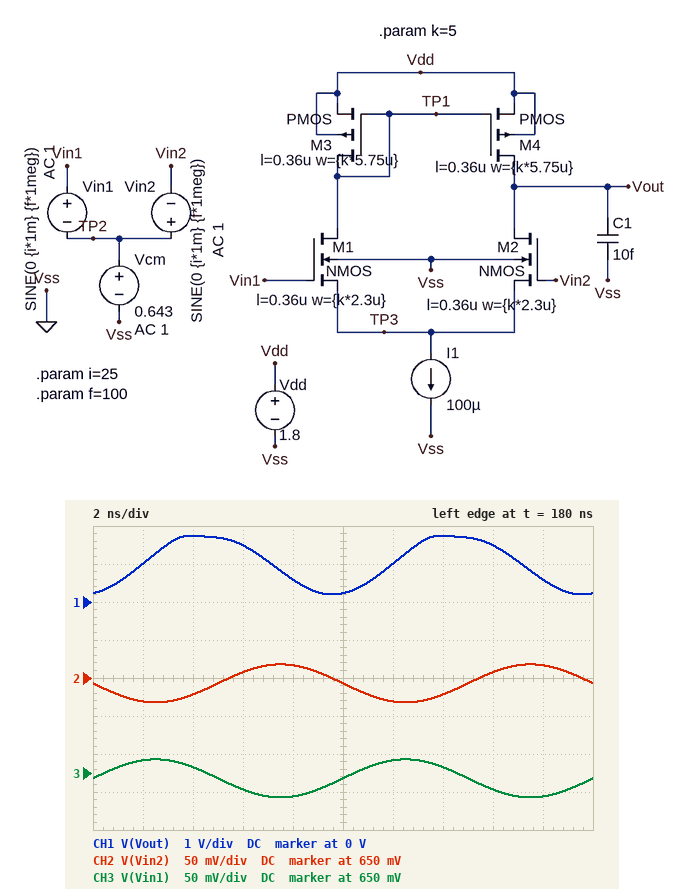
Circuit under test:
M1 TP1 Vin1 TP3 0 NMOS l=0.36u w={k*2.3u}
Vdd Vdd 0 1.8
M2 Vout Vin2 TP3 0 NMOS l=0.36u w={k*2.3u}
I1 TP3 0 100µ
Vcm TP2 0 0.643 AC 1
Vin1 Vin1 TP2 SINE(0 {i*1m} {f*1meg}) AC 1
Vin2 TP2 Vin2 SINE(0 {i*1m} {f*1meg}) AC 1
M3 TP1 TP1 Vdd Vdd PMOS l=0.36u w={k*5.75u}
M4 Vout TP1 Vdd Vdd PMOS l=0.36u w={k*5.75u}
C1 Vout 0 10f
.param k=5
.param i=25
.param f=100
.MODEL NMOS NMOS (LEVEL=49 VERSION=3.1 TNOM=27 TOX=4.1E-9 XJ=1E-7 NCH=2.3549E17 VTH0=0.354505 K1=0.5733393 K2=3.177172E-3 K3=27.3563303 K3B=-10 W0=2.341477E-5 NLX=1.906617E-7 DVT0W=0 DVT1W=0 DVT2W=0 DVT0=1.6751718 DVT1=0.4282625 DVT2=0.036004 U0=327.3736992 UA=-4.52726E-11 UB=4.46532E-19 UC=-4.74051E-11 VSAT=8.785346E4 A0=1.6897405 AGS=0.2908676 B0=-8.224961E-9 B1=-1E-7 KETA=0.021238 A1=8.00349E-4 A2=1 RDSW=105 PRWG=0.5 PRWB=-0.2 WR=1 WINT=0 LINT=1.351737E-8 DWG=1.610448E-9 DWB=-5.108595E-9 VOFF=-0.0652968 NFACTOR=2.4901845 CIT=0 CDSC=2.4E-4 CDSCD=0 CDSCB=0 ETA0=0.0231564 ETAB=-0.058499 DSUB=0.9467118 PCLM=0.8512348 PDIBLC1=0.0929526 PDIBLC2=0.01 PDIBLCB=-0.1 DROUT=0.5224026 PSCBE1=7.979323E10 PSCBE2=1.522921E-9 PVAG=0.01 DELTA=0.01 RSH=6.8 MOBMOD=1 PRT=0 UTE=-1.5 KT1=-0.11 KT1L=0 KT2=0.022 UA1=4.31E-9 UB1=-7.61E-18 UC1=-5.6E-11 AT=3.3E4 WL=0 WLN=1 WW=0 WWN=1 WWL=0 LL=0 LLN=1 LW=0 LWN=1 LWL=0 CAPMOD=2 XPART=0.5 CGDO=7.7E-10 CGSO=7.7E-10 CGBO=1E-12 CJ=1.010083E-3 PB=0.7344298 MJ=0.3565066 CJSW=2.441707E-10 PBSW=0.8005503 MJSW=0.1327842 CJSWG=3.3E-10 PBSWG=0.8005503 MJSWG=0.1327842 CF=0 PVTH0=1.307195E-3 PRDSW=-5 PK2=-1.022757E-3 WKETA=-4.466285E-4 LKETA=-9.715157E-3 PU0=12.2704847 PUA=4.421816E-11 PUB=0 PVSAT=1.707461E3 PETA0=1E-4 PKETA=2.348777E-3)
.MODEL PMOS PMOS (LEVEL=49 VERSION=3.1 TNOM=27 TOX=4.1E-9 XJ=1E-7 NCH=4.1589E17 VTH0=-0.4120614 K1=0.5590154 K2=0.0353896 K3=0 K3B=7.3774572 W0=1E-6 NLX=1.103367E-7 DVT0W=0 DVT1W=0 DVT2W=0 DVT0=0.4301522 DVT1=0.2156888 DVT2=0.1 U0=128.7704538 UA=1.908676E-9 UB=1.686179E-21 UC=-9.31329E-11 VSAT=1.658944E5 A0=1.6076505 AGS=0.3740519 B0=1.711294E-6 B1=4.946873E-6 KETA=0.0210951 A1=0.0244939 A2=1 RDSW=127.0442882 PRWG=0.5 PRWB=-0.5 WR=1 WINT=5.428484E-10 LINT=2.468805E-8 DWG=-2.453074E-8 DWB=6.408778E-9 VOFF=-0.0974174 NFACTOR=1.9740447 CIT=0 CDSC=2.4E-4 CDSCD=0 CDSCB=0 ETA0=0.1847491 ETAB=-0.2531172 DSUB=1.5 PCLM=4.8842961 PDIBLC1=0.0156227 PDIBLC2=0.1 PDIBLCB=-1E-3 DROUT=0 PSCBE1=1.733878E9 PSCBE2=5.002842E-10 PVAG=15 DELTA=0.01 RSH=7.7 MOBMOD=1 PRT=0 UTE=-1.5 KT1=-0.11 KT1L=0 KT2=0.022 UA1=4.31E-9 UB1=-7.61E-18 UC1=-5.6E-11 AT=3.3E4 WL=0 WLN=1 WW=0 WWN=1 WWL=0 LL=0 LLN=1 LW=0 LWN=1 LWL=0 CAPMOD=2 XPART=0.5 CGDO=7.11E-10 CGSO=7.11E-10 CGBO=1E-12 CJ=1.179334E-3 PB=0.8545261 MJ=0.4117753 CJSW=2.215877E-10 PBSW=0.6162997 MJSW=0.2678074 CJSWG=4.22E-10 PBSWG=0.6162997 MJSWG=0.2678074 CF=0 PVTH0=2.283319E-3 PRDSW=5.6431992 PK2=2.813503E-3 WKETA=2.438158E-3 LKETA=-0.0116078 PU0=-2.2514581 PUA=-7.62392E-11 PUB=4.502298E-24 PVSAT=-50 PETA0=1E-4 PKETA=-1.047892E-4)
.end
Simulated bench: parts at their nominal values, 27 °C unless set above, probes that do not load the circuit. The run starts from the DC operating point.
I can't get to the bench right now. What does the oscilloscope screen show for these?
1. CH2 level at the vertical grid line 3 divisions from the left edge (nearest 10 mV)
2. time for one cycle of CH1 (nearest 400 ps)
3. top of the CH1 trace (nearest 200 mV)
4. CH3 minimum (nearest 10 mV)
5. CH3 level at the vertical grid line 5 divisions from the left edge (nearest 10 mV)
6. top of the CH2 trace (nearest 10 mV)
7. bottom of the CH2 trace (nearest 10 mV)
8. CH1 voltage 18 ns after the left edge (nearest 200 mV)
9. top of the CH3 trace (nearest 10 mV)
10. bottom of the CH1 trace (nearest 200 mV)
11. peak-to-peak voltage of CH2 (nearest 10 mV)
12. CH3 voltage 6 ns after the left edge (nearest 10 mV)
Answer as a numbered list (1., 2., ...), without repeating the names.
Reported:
1. 660 mV
2. 10.0 ns
3. 1.8 V
4. 620 mV
5. 640 mV
6. 670 mV
7. 620 mV
8. 600 mV
9. 670 mV
10. 200 mV
11. 50 mV
12. 630 mV
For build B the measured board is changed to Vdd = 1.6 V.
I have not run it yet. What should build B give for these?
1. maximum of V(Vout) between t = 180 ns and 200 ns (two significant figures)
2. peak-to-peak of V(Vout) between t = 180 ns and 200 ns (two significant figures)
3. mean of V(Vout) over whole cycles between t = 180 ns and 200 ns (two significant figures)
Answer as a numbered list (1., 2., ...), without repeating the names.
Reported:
1. 1.5 V
2. 1.4 V
3. 860 mV
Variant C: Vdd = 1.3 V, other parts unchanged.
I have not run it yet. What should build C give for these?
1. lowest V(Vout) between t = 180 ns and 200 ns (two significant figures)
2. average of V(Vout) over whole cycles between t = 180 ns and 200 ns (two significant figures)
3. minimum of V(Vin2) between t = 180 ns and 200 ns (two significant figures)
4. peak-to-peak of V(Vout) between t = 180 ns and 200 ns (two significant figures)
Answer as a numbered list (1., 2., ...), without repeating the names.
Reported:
1. 73 mV
2. 680 mV
3. 620 mV
4. 1.2 V
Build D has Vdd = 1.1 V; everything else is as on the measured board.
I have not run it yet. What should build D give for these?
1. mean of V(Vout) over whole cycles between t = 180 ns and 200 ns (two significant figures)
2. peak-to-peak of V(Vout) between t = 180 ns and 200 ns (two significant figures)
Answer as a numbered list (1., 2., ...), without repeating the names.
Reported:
1. 560 mV
2. 990 mV
